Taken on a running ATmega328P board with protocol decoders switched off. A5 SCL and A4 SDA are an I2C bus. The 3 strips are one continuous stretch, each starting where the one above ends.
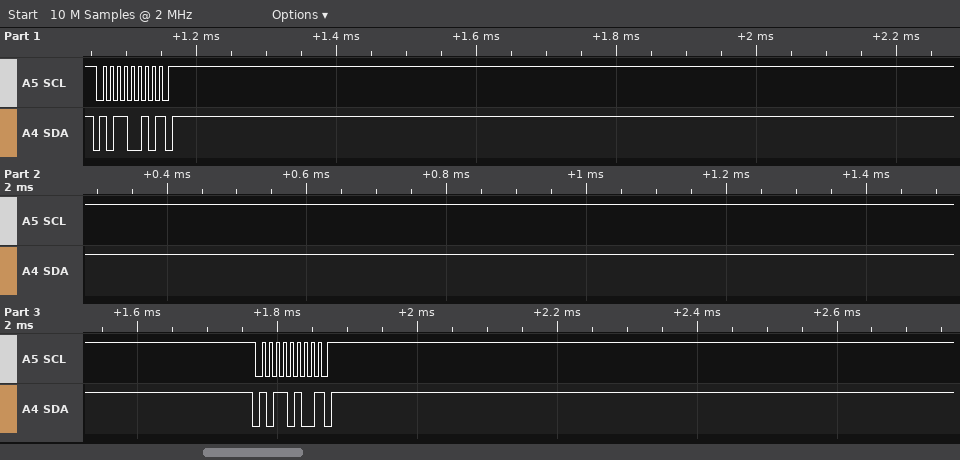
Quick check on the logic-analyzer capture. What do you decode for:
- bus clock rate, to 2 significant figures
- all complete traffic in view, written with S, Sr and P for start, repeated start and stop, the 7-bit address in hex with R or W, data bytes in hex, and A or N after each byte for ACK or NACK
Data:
100 kHz
S 59W N P S 5AW N P
